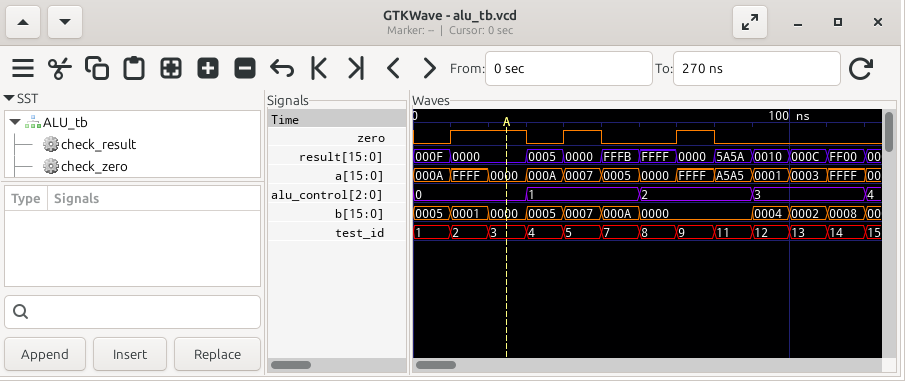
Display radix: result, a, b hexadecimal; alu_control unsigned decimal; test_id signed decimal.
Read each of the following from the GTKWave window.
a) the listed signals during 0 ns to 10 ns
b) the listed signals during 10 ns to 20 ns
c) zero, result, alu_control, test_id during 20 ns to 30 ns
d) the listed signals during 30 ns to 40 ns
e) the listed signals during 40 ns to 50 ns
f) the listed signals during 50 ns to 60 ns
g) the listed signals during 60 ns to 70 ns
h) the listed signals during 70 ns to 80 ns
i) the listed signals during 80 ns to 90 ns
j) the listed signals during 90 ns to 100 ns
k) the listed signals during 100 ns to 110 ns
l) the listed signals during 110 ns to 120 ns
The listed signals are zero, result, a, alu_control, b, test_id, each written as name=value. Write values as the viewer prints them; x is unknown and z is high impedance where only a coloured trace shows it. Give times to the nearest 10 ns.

zero=0, result=000F, a=000A, alu_control=0, b=0005, test_id=1
zero=1, result=0000, a=FFFF, alu_control=0, b=0001, test_id=2
zero=1, result=0000, alu_control=0, test_id=3
zero=0, result=0005, a=000A, alu_control=1, b=0005, test_id=4
zero=1, result=0000, a=0007, alu_control=1, b=0007, test_id=5
zero=0, result=FFFB, a=0005, alu_control=1, b=000A, test_id=7
zero=0, result=FFFF, a=0000, alu_control=2, b=0000, test_id=8
zero=1, result=0000, a=FFFF, alu_control=2, b=0000, test_id=9
zero=0, result=5A5A, a=A5A5, alu_control=2, b=0000, test_id=11
zero=0, result=0010, a=0001, alu_control=3, b=0004, test_id=12
zero=0, result=000C, a=0003, alu_control=3, b=0002, test_id=13
zero=0, result=FF00, a=FFFF, alu_control=3, b=0008, test_id=14
